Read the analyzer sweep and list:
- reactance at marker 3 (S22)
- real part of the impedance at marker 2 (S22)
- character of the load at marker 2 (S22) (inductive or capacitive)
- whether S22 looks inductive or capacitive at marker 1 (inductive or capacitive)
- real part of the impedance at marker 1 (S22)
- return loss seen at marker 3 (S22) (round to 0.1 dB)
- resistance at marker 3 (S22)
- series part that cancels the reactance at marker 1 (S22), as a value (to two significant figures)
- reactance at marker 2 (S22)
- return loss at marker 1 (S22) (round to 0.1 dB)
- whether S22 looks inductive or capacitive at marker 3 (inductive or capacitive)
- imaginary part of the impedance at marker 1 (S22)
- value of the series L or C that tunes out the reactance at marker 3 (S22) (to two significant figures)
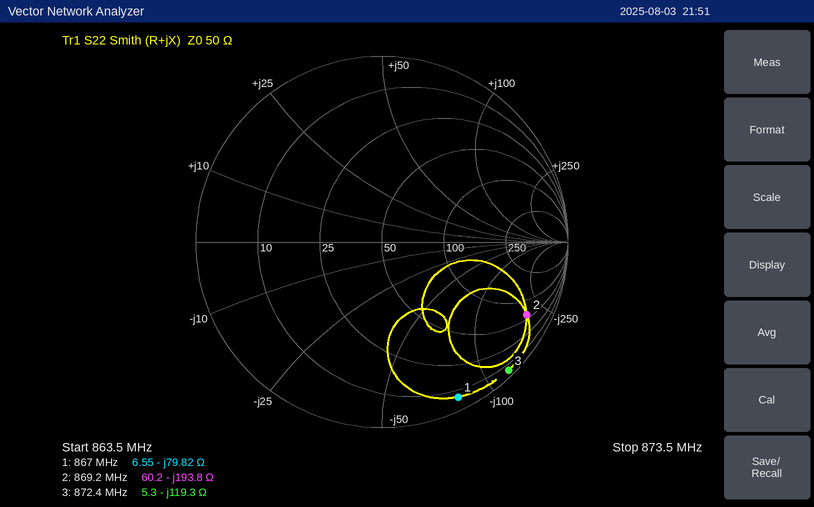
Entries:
-119.3 Ω
60.2 Ω
capacitive
capacitive
6.55 Ω
0.3 dB
5.3 Ω
15 nH
-193.8 Ω
0.6 dB
capacitive
-79.82 Ω
22 nH
